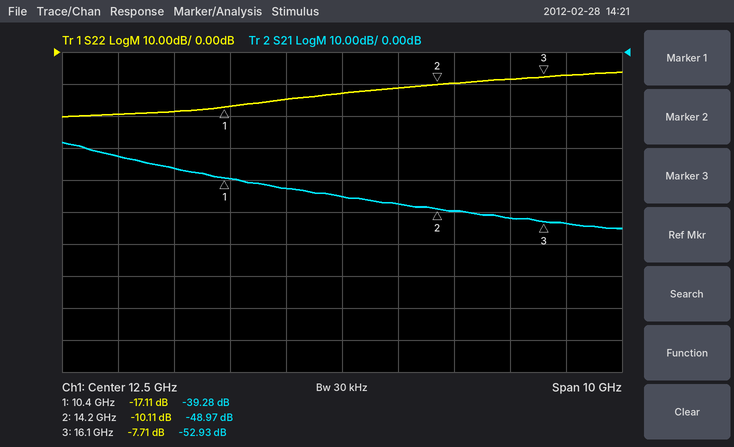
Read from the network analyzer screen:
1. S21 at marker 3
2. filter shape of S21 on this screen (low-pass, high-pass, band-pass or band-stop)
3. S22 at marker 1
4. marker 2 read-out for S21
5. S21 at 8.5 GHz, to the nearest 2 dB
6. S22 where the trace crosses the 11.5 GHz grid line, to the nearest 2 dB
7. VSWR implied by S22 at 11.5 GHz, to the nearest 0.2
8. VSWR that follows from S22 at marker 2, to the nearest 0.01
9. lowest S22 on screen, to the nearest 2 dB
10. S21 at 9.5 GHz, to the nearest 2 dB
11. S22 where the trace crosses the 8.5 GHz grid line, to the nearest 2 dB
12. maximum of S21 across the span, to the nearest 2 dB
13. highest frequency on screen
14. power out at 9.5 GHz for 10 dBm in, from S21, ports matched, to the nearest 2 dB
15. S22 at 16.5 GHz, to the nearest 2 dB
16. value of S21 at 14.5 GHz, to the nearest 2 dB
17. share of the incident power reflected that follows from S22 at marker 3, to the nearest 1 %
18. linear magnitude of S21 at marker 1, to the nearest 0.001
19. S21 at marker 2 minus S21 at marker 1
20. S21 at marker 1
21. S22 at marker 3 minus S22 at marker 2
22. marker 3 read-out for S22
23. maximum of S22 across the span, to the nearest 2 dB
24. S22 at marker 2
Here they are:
-52.93 dB
low-pass
-17.11 dB
-48.97 dB
-32 dB
-14 dB
1.4
1.91
-20 dB
-36 dB
-20 dB
-28 dB
17.5 GHz
-26 dBm
-8 dB
-50 dB
17 %
0.011
-9.69 dB
-39.28 dB
2.40 dB
-7.71 dB
-6 dB
-10.11 dB
